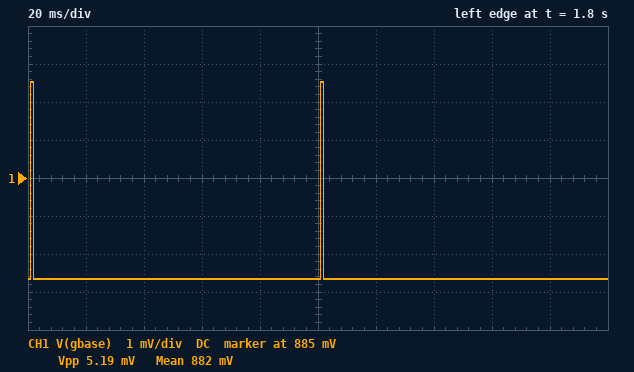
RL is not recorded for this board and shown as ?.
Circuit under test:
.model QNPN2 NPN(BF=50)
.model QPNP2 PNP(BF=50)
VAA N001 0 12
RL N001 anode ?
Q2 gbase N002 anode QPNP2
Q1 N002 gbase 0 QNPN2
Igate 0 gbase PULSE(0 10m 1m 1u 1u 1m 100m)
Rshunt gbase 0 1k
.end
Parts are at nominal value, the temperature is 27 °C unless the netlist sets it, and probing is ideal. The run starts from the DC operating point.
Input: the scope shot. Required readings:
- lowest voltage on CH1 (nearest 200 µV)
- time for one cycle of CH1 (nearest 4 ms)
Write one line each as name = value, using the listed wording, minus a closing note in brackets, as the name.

lowest voltage on CH1 = 882.4 mV
time for one cycle of CH1 = 100 ms
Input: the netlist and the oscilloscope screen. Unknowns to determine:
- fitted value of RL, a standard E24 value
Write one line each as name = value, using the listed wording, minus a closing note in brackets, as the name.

fitted value of RL, a standard E24 value = 240 Ω
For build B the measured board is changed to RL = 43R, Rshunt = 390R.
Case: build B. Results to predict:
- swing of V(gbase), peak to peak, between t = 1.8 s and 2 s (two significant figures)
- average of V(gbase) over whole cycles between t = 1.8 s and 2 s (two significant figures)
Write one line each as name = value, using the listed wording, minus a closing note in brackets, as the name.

swing of V(gbase), peak to peak, between t = 1.8 s and 2 s = 1.0 mV
average of V(gbase) over whole cycles between t = 1.8 s and 2 s = 930 mV
